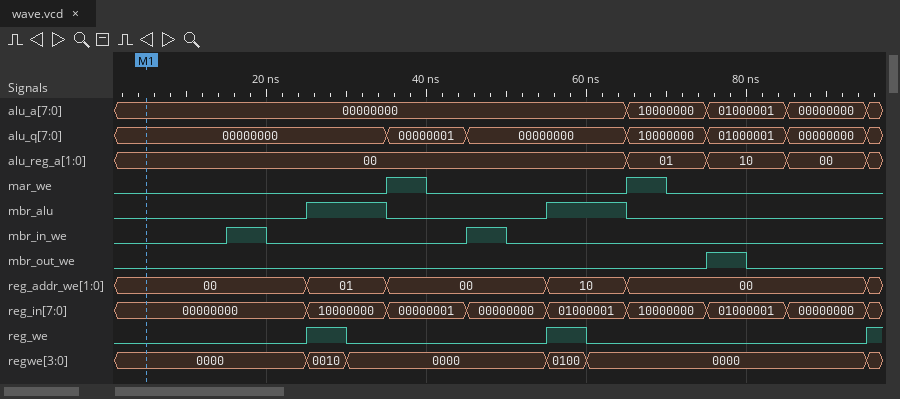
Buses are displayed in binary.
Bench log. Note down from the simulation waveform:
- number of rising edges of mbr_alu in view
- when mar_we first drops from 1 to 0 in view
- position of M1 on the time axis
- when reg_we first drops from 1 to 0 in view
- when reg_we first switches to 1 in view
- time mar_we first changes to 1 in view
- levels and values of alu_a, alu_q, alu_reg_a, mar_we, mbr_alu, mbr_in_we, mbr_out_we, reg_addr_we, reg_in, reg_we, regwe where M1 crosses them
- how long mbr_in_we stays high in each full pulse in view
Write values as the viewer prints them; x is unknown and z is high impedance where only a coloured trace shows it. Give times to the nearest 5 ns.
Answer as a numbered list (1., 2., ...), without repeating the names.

1. 2
2. 40 ns
3. 5 ns
4. 30 ns
5. 25 ns
6. 35 ns
7. alu_a=00000000, alu_q=00000000, alu_reg_a=00, mar_we=0, mbr_alu=0, mbr_in_we=0, mbr_out_we=0, reg_addr_we=00, reg_in=00000000, reg_we=0, regwe=0000
8. 5 ns, 5 ns
